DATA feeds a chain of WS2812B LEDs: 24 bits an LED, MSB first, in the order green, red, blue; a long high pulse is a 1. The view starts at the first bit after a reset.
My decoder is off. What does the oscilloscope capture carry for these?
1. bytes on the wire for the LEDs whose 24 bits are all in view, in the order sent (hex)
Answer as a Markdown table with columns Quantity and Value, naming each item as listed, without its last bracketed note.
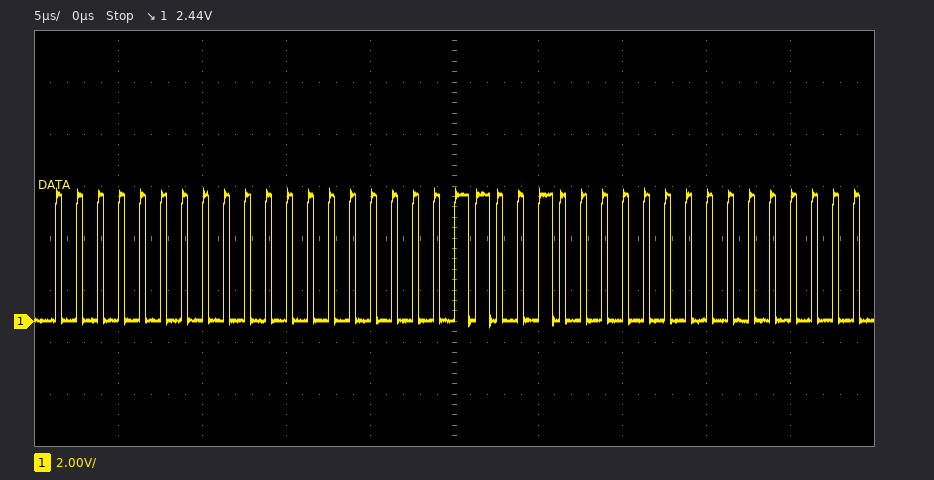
| Quantity | Value |
|---|---|
| bytes on the wire for the LEDs whose 24 bits are all in view, in the order sent | 00 00 19 |
